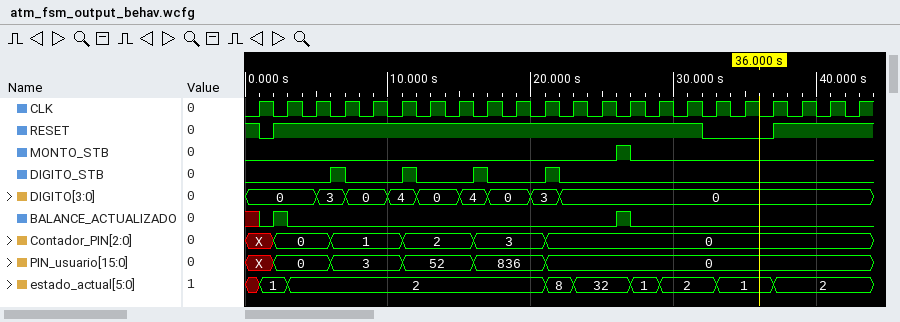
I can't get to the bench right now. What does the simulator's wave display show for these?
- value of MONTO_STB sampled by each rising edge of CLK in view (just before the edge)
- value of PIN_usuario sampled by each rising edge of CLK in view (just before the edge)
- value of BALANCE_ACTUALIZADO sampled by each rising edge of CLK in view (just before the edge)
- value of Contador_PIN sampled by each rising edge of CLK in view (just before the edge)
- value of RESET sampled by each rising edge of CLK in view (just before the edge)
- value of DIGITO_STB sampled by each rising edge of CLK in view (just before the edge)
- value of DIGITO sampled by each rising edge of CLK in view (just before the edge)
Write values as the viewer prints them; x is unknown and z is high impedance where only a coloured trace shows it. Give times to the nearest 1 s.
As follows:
0 0 0 0 0 0 0 0 0 0 0 0 0 1 0 0 0 0 0 0 0 0
X, 0, 0, 3, 3, 3, 52, 52, 836, 836, 836, 0, 0, 0, 0, 0, 0, 0, 0, 0, 0, 0
x 1 0 0 0 0 0 0 0 0 0 0 0 1 0 0 0 0 0 0 0 0
X, 0, 0, 1, 1, 1, 2, 2, 3, 3, 3, 0, 0, 0, 0, 0, 0, 0, 0, 0, 0, 0
1 1 1 1 1 1 1 1 1 1 1 1 1 1 1 1 0 0 0 1 1 1
0 0 0 1 0 0 0 0 1 0 0 0 0 0 0 0 0 0 0 0 0 0
0, 0, 0, 3, 0, 4, 0, 0, 4, 0, 3, 0, 0, 0, 0, 0, 0, 0, 0, 0, 0, 0
